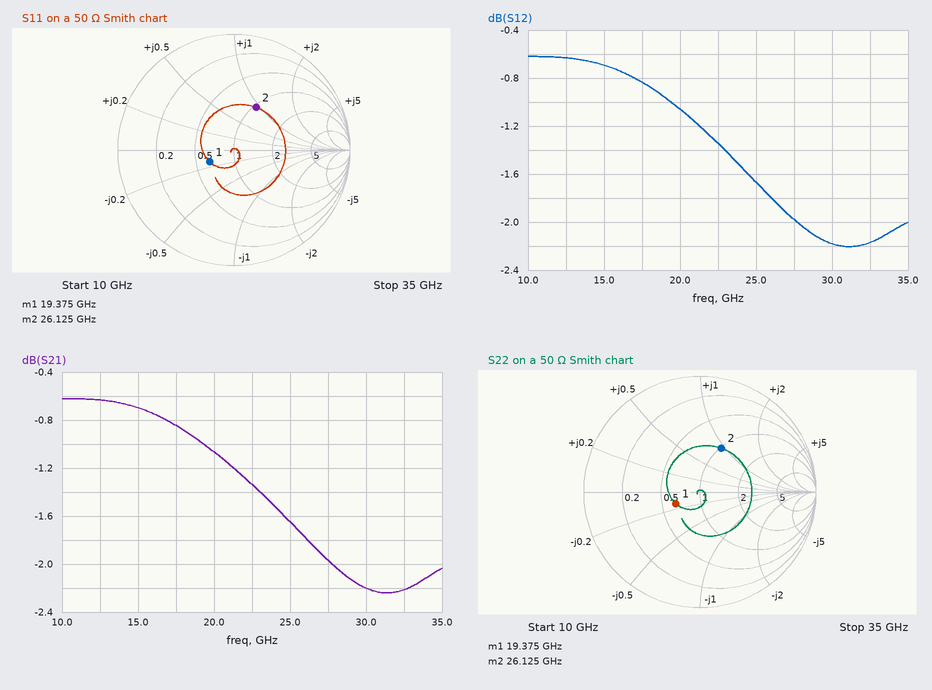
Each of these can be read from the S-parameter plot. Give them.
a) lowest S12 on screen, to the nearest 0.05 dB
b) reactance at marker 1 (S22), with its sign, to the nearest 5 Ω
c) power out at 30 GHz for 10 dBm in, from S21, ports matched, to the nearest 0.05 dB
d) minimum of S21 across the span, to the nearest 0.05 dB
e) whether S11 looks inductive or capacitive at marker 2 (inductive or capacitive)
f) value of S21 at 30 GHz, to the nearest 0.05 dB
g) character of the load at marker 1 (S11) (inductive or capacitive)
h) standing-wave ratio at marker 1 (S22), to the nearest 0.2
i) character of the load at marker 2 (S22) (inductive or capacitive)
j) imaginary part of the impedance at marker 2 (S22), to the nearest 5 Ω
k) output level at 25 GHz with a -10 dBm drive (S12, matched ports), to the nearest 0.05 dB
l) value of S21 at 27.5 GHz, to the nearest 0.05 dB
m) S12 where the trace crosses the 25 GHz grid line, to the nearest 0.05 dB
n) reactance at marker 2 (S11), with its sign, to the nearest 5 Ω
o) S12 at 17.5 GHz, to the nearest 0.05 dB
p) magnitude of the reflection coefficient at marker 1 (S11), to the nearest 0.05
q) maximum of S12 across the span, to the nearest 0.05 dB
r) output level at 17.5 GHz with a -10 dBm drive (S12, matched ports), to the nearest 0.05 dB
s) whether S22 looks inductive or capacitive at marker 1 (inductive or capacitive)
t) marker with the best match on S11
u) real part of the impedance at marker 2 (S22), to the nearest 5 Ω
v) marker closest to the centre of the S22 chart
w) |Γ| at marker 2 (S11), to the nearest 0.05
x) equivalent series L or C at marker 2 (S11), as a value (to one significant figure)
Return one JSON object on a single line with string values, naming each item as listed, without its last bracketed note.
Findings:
{"lowest S12 on screen, to the nearest 0.05 dB": "-2.20 dB", "reactance at marker 1 (S22), with its sign, to the nearest 5 Ω": "-5 Ω", "power out at 30 GHz for 10 dBm in, from S21, ports matched, to the nearest 0.05 dB": "7.80 dBm", "minimum of S21 across the span, to the nearest 0.05 dB": "-2.25 dB", "whether S11 looks inductive or capacitive at marker 2": "inductive", "value of S21 at 30 GHz, to the nearest 0.05 dB": "-2.20 dB", "character of the load at marker 1 (S11)": "capacitive", "standing-wave ratio at marker 1 (S22), to the nearest 0.2": "1.6", "character of the load at marker 2 (S22)": "inductive", "imaginary part of the impedance at marker 2 (S22), to the nearest 5 Ω": "+45 Ω", "output level at 25 GHz with a -10 dBm drive (S12, matched ports), to the nearest 0.05 dB": "-11.65 dBm", "value of S21 at 27.5 GHz, to the nearest 0.05 dB": "-1.95 dB", "S12 where the trace crosses the 25 GHz grid line, to the nearest 0.05 dB": "-1.65 dB", "reactance at marker 2 (S11), with its sign, to the nearest 5 Ω": "+45 Ω", "S12 at 17.5 GHz, to the nearest 0.05 dB": "-0.85 dB", "magnitude of the reflection coefficient at marker 1 (S11), to the nearest 0.05": "0.25", "maximum of S12 across the span, to the nearest 0.05 dB": "-0.60 dB", "output level at 17.5 GHz with a -10 dBm drive (S12, matched ports), to the nearest 0.05 dB": "-10.85 dBm", "whether S22 looks inductive or capacitive at marker 1": "capacitive", "marker with the best match on S11": "marker 1", "real part of the impedance at marker 2 (S22), to the nearest 5 Ω": "50 Ω", "marker closest to the centre of the S22 chart": "marker 1", "|Γ| at marker 2 (S11), to the nearest 0.05": "0.40", "equivalent series L or C at marker 2 (S11), as a value": "300 pH"}
